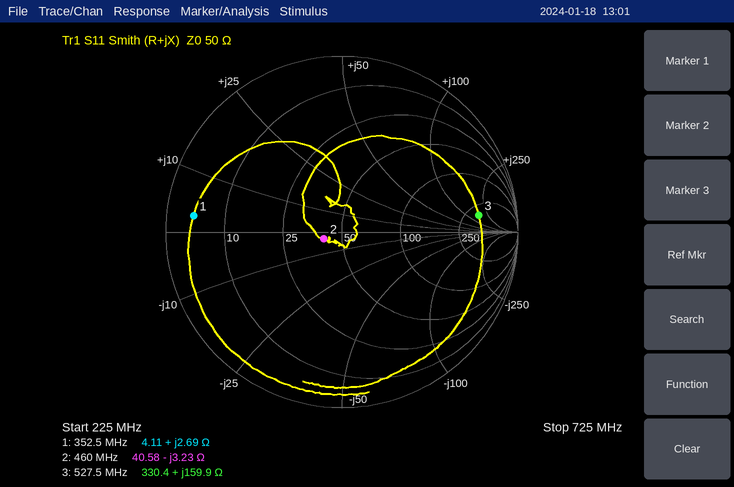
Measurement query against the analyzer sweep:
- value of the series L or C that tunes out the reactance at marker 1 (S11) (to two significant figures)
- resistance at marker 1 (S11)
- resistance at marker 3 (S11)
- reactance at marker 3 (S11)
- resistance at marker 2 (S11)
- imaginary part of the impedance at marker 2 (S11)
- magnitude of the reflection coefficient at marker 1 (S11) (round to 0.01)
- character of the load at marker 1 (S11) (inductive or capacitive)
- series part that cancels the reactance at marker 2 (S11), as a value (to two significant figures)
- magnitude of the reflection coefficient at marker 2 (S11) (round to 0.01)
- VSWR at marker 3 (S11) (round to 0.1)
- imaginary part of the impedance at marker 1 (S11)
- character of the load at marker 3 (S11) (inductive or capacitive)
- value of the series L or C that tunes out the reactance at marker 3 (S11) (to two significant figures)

170 pF
4.11 Ω
330.4 Ω
+159.9 Ω
40.58 Ω
-3.23 Ω
0.85
inductive
1.1 nH
0.11
8.2
+2.69 Ω
inductive
1.9 pF
